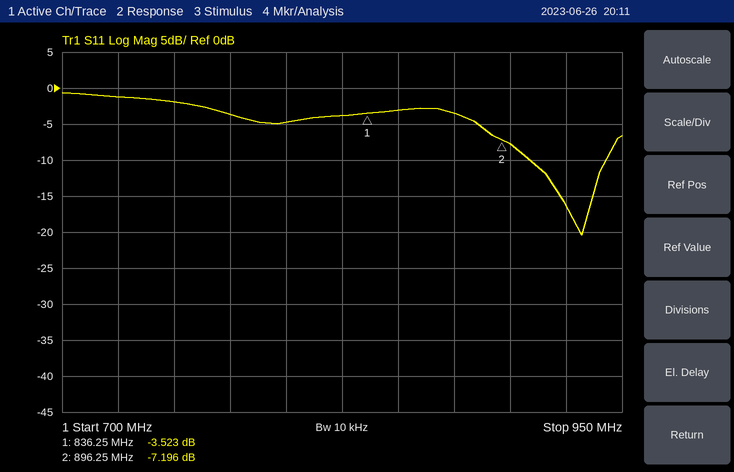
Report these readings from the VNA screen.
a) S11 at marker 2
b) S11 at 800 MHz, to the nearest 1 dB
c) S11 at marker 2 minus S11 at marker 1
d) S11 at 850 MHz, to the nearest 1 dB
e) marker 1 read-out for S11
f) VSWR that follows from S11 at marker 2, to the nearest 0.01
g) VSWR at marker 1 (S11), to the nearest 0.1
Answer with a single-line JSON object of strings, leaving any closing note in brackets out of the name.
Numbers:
{"S11 at marker 2": "-7.196 dB", "S11 at 800 MHz, to the nearest 1 dB": "-5 dB", "S11 at marker 2 minus S11 at marker 1": "-3.673 dB", "S11 at 850 MHz, to the nearest 1 dB": "-3 dB", "marker 1 read-out for S11": "-3.523 dB", "VSWR that follows from S11 at marker 2, to the nearest 0.01": "2.55", "VSWR at marker 1 (S11), to the nearest 0.1": "5.0"}
